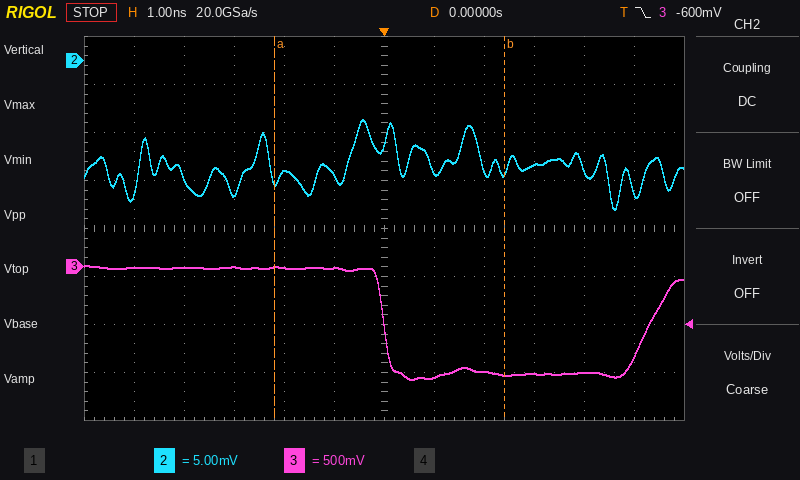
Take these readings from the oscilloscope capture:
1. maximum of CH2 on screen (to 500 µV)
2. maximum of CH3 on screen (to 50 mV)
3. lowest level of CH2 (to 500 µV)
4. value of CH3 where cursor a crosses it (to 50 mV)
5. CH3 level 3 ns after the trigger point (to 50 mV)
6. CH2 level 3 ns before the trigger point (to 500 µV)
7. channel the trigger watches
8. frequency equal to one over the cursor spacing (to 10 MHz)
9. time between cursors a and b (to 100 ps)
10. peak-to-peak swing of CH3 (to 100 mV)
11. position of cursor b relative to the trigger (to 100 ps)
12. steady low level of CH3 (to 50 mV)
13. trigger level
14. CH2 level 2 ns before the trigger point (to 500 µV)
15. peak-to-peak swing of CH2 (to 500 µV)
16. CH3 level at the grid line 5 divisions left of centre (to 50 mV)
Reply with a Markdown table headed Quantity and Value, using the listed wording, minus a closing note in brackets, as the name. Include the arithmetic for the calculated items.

| Quantity | Value |
|---|---|
| maximum of CH2 on screen | -6.0 mV |
| maximum of CH3 on screen | 0 mV |
| lowest level of CH2 | -15.5 mV |
| value of CH3 where cursor a crosses it | 0 mV |
| CH3 level 3 ns after the trigger point | -1.10 V |
| CH2 level 3 ns before the trigger point | -14.0 mV |
| channel the trigger watches | CH3 |
| frequency equal to one over the cursor spacing | 1 / 4.6 ns ≈ 220 MHz |
| time between cursors a and b | 4.6 ns |
| peak-to-peak swing of CH3 | 1.20 V |
| position of cursor b relative to the trigger | +2.4 ns |
| steady low level of CH3 | -1.10 V |
| trigger level | -600 mV |
| CH2 level 2 ns before the trigger point | -11.5 mV |
| peak-to-peak swing of CH2 | -6.0 mV − (-15.5 mV) = 9.5 mV |
| CH3 level at the grid line 5 divisions left of centre | 0 mV |
